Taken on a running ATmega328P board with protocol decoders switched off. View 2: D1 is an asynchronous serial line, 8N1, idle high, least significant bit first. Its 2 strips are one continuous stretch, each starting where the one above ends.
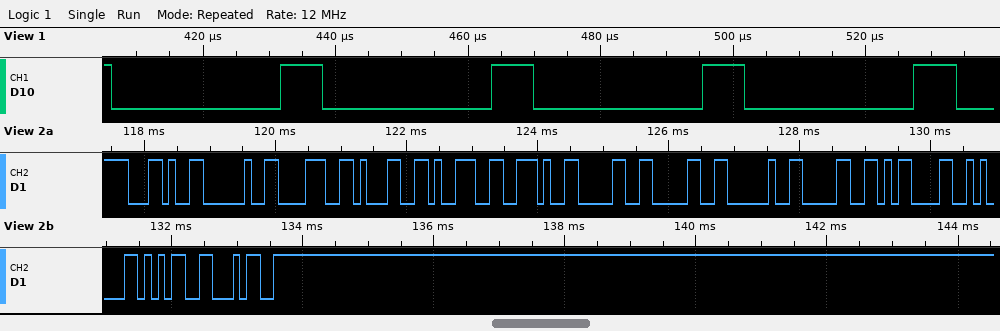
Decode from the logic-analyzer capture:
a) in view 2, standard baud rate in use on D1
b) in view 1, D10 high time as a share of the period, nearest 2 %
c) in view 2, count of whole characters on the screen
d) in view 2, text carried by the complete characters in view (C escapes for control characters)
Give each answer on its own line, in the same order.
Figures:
9600 baud
20 %
14
", 819.00 0\r\n54"
